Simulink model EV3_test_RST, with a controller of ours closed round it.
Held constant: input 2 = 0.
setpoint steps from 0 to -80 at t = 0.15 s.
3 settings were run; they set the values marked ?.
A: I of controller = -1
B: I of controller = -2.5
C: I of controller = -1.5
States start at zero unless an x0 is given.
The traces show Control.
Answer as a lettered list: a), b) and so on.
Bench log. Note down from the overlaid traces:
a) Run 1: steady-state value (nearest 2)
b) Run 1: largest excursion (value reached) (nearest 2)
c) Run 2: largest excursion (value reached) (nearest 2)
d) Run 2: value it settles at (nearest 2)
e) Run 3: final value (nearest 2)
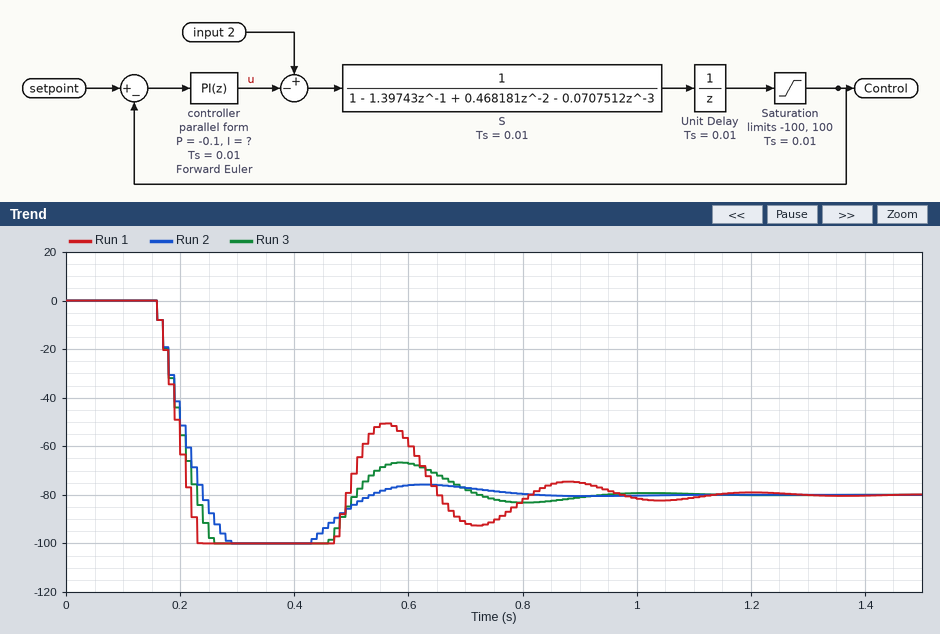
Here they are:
a) -80
b) -100
c) -100
d) -80
e) -80
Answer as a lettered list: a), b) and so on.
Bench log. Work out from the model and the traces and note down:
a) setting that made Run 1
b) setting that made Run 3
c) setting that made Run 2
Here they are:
a) B
b) C
c) A
